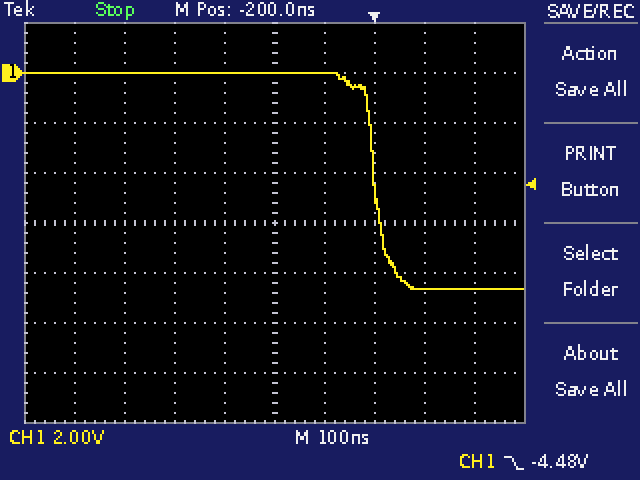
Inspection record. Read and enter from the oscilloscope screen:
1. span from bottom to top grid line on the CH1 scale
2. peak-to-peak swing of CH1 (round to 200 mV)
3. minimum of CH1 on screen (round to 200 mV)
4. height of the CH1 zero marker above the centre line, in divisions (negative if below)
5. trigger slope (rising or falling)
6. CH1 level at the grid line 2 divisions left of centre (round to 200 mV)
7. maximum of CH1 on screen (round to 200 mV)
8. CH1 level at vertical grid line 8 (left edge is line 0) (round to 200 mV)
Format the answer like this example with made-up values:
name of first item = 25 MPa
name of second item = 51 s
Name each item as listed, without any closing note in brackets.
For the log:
span from bottom to top grid line on the CH1 scale = 16 V
peak-to-peak swing of CH1 = 8.6 V
minimum of CH1 on screen = -8.6 V
height of the CH1 zero marker above the centre line, in divisions = +3.0 div
trigger slope = falling
CH1 level at the grid line 2 divisions left of centre = 0.0 V
maximum of CH1 on screen = 0.0 V
CH1 level at vertical grid line 8 (left edge is line 0) = -8.6 V
